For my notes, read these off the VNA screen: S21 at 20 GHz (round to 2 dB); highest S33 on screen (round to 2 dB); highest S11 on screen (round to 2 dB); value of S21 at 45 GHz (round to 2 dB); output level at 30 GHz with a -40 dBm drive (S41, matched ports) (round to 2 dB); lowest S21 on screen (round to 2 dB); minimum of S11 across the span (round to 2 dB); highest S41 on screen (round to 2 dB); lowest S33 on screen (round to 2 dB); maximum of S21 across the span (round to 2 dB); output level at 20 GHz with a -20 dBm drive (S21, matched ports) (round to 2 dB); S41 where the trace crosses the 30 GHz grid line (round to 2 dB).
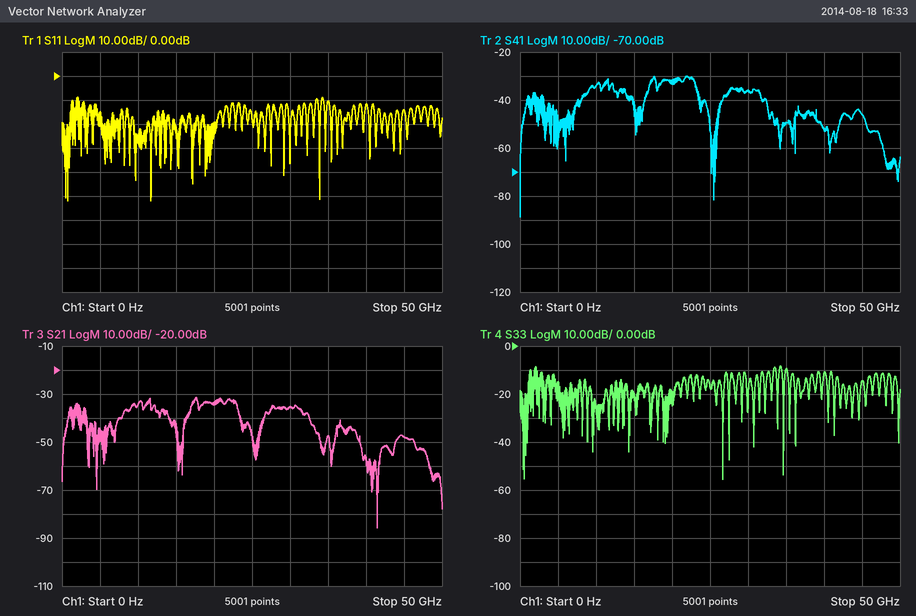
-34 dB
-8 dB
-8 dB
-48 dB
-76 dBm
-86 dB
-52 dB
-30 dB
-56 dB
-32 dB
-54 dBm
-36 dB
